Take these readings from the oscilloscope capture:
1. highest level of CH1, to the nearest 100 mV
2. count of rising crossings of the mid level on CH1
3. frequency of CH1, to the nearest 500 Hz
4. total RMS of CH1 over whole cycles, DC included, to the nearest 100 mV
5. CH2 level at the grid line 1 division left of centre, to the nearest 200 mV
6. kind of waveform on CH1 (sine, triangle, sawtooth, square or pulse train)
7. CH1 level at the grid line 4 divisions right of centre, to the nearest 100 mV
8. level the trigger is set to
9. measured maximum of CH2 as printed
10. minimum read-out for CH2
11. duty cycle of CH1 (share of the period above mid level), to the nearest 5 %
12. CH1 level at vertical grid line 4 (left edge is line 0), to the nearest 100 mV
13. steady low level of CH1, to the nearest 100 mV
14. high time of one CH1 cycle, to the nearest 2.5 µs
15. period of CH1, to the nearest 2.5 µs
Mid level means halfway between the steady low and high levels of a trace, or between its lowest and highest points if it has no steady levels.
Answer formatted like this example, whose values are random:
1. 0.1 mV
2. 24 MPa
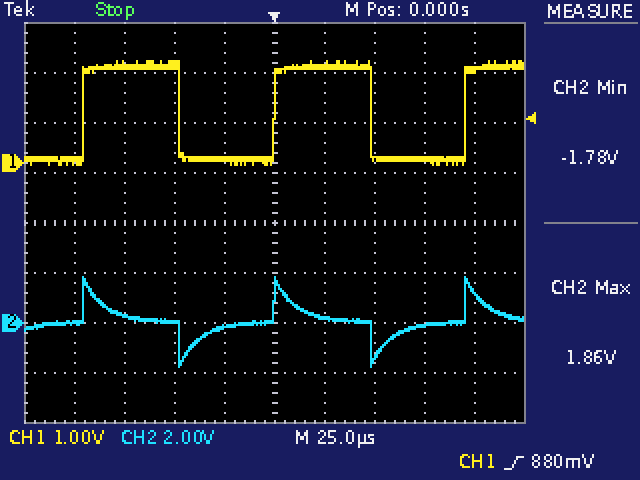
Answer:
1. 2.0 V
2. 3
3. 10.5 kHz
4. 1.4 V
5. -200 mV
6. square
7. 1.9 V
8. 880 mV
9. 1.86 V
10. -1.78 V
11. 50 %
12. 100 mV
13. 100 mV
14. 47.5 µs
15. 95.0 µs
